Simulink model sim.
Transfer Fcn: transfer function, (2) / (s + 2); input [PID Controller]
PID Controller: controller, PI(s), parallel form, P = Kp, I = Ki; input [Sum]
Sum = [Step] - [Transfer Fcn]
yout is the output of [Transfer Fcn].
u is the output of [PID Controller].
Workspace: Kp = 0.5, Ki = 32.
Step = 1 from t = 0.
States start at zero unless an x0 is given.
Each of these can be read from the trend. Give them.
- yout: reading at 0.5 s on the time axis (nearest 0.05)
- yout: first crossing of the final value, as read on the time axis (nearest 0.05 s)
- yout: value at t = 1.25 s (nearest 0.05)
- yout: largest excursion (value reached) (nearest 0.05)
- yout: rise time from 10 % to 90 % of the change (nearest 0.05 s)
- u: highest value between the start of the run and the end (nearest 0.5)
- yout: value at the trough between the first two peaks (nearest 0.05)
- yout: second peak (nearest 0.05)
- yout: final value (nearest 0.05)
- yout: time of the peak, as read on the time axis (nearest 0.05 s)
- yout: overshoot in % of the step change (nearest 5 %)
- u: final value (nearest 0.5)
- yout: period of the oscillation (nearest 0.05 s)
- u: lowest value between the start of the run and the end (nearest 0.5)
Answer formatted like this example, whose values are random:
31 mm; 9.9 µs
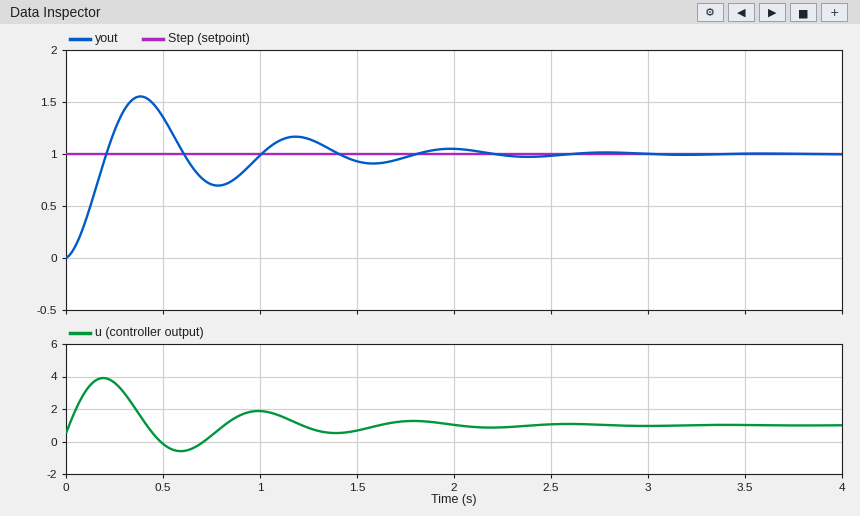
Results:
1.35; 0.20 s; 1.15; 1.55; 0.15 s; 4.0; 0.70; 1.15; 1.00; 0.40 s; 55 %; 1.0; 0.80 s; -0.5
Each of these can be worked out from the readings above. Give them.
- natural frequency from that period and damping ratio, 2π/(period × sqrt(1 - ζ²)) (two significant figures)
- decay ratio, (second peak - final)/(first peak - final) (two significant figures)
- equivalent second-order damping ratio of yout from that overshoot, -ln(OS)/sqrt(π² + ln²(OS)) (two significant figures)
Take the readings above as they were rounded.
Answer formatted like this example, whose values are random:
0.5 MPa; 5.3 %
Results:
8.0 rad/s; 0.27; 0.19
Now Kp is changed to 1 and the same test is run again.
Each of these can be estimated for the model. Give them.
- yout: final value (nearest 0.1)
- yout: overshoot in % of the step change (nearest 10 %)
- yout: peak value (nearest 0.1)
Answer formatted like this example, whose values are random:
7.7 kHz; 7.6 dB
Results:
1.0; 50 %; 1.5
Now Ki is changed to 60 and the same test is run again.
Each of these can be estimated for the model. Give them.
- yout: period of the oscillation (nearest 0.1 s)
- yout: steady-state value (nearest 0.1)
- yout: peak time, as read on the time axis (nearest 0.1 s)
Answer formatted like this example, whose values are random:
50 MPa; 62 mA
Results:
0.6 s; 1.0; 0.3 s
